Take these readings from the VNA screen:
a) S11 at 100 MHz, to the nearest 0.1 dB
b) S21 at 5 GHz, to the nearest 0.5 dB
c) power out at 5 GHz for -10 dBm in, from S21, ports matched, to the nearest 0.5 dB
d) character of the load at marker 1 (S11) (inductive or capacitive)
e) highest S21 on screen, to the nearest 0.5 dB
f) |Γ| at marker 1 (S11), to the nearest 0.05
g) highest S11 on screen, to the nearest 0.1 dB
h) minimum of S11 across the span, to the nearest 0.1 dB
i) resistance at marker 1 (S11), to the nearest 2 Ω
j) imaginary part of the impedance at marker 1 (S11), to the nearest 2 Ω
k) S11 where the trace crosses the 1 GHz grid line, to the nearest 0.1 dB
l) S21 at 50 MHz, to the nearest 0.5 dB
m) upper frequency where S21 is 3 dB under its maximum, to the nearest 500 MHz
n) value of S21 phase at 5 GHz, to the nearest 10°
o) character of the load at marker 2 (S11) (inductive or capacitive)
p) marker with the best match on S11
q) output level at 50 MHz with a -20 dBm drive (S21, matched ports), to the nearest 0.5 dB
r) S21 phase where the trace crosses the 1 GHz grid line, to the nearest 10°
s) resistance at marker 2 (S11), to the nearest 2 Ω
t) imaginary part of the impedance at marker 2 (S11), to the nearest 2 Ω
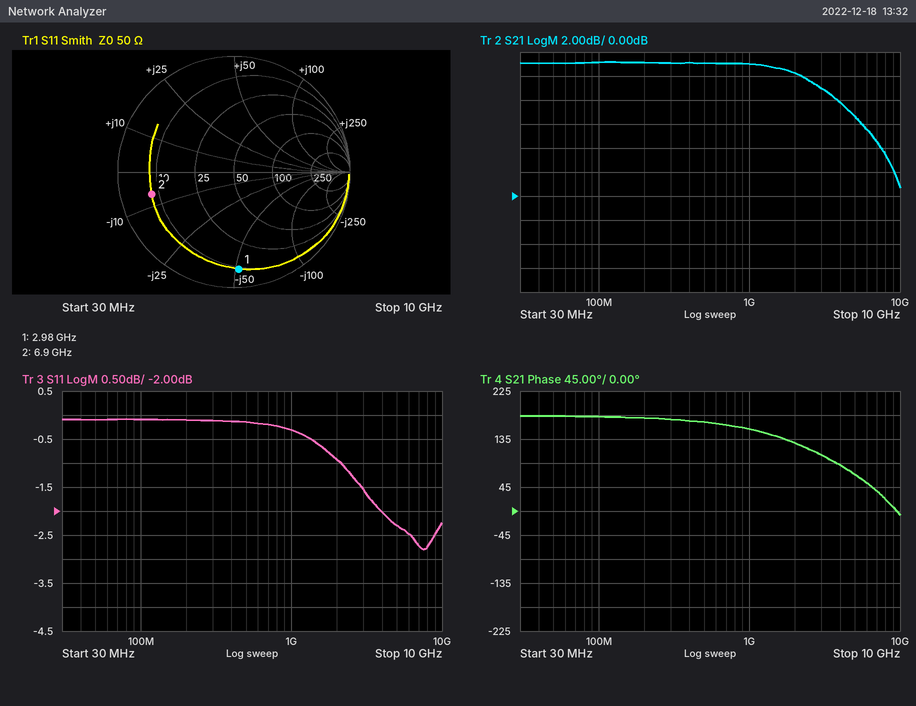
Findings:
-0.1 dB
6.5 dB
-3.5 dBm
capacitive
11.0 dB
0.85
-0.1 dB
-2.8 dB
10 Ω
-52 Ω
-0.3 dB
11.0 dB
3.5 GHz
70°
capacitive
marker 2
-9.0 dBm
150°
8 Ω
-6 Ω
